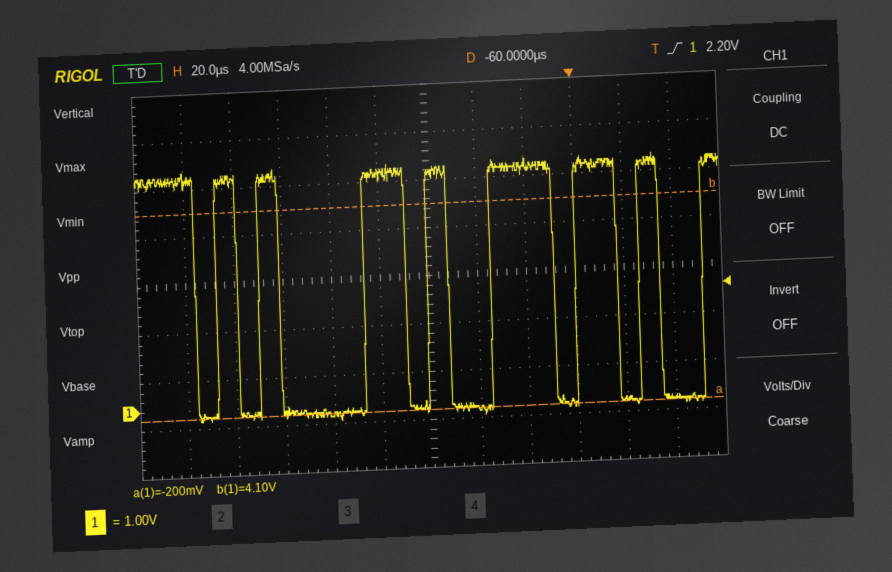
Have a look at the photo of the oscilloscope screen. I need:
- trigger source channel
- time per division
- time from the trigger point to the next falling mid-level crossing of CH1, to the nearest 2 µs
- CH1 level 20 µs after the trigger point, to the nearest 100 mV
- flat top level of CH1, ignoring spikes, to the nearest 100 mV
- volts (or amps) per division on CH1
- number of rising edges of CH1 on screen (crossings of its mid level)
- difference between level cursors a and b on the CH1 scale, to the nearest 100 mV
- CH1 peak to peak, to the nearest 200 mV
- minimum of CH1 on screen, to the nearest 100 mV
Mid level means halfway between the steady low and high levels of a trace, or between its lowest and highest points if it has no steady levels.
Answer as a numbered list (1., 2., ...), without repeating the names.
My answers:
1. CH1
2. 20 µs
3. 18 µs
4. -100 mV
5. 4.8 V
6. 1 V
7. 8
8. 4.3 V
9. 5.2 V
10. -300 mV
